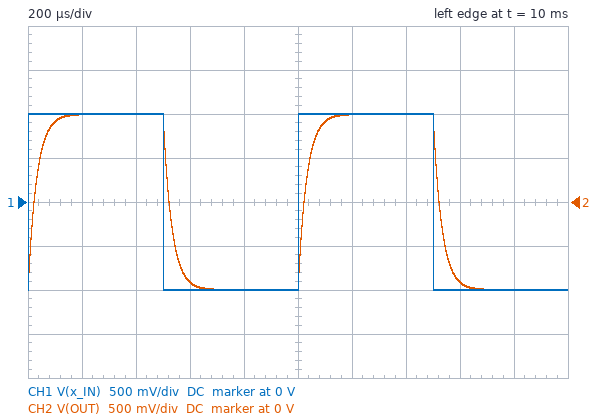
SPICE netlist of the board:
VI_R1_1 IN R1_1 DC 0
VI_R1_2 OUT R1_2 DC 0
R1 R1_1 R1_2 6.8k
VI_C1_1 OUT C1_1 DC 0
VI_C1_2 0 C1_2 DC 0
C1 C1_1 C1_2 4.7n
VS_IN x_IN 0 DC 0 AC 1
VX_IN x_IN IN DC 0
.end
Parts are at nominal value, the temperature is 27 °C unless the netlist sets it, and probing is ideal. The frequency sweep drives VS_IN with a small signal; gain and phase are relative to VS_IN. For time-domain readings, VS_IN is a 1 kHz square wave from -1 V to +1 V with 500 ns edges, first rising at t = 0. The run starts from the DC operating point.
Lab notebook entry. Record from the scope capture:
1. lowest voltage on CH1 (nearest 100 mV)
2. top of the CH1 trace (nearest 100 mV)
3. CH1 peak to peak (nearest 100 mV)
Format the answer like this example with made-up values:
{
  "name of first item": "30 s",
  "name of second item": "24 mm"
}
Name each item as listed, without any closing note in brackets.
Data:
{
  "lowest voltage on CH1": "-1.0 V",
  "top of the CH1 trace": "1.0 V",
  "CH1 peak to peak": "2.0 V"
}
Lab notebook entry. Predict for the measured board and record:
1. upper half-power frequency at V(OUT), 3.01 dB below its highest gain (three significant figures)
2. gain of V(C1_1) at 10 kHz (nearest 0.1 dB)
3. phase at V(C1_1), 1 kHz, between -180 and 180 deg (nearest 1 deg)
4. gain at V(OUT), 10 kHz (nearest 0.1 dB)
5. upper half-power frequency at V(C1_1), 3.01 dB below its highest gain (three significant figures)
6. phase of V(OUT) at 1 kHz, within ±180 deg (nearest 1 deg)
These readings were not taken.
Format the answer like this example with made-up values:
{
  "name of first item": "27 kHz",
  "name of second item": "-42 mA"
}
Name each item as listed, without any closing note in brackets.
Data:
{
  "upper half-power frequency at V(OUT), 3.01 dB below its highest gain": "4.98 kHz",
  "gain of V(C1_1) at 10 kHz": "-7.0 dB",
  "phase at V(C1_1), 1 kHz, between -180 and 180 deg": "-11 deg",
  "gain at V(OUT), 10 kHz": "-7.0 dB",
  "upper half-power frequency at V(C1_1), 3.01 dB below its highest gain": "4.98 kHz",
  "phase of V(OUT) at 1 kHz, within ±180 deg": "-11 deg"
}
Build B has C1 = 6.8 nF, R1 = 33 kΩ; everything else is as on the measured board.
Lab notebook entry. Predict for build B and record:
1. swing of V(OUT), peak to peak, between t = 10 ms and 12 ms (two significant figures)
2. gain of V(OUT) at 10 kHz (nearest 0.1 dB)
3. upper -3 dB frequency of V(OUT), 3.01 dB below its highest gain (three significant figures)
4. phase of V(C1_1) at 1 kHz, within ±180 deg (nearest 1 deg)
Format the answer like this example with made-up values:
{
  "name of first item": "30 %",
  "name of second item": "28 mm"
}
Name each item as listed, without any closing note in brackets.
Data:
{
  "swing of V(OUT), peak to peak, between t = 10 ms and 12 ms": "1.6 V",
  "gain of V(OUT) at 10 kHz": "-23.0 dB",
  "upper -3 dB frequency of V(OUT), 3.01 dB below its highest gain": "709 Hz",
  "phase of V(C1_1) at 1 kHz, within ±180 deg": "-55 deg"
}
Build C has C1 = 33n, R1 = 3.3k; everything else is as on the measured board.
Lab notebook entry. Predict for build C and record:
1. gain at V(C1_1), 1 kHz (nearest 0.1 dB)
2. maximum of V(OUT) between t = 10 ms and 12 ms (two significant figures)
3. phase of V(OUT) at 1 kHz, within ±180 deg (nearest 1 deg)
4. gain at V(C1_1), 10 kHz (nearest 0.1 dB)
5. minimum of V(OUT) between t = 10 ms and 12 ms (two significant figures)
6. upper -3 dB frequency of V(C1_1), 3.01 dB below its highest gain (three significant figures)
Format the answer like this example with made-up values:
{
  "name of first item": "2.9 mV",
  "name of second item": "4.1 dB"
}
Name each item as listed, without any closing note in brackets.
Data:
{
  "gain at V(C1_1), 1 kHz": "-1.7 dB",
  "maximum of V(OUT) between t = 10 ms and 12 ms": "980 mV",
  "phase of V(OUT) at 1 kHz, within ±180 deg": "-34 deg",
  "gain at V(C1_1), 10 kHz": "-16.8 dB",
  "minimum of V(OUT) between t = 10 ms and 12 ms": "-980 mV",
  "upper -3 dB frequency of V(C1_1), 3.01 dB below its highest gain": "1.46 kHz"
}
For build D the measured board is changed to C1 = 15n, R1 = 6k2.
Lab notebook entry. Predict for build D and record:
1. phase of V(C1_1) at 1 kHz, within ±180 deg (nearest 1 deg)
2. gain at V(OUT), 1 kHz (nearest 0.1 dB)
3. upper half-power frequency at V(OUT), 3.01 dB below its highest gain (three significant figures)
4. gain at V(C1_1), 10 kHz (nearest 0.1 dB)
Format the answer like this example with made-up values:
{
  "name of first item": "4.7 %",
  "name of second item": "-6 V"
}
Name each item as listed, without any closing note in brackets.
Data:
{
  "phase of V(C1_1) at 1 kHz, within ±180 deg": "-30 deg",
  "gain at V(OUT), 1 kHz": "-1.3 dB",
  "upper half-power frequency at V(OUT), 3.01 dB below its highest gain": "1.71 kHz",
  "gain at V(C1_1), 10 kHz": "-15.5 dB"
}
